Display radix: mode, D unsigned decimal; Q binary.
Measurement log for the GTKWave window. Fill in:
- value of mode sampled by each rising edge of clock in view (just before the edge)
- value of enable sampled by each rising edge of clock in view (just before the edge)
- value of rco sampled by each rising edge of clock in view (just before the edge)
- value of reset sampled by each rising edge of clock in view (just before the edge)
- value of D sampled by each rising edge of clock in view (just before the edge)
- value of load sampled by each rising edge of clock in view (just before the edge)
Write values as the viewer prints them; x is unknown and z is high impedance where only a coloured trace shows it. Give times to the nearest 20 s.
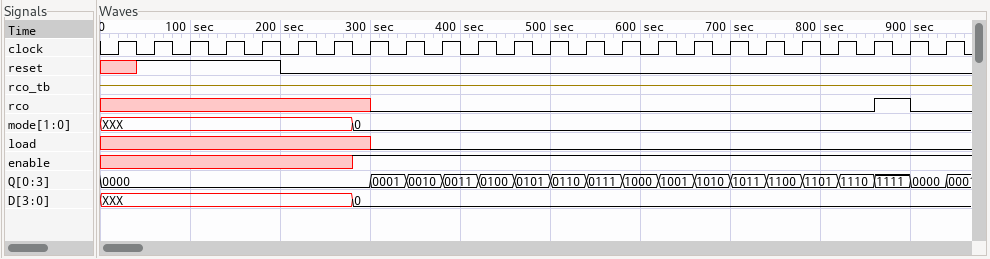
XXX, XXX, XXX, XXX, XXX, XXX, XXX, 0, 0, 0, 0, 0, 0, 0, 0, 0, 0, 0, 0, 0, 0, 0, 0, 0
x x x x x x x 1 1 1 1 1 1 1 1 1 1 1 1 1 1 1 1 1
x x x x x x x x 0 0 0 0 0 0 0 0 0 0 0 0 0 0 1 0
x 1 1 1 1 0 0 0 0 0 0 0 0 0 0 0 0 0 0 0 0 0 0 0
XXX, XXX, XXX, XXX, XXX, XXX, XXX, 0, 0, 0, 0, 0, 0, 0, 0, 0, 0, 0, 0, 0, 0, 0, 0, 0
x x x x x x x x 0 0 0 0 0 0 0 0 0 0 0 0 0 0 0 0
